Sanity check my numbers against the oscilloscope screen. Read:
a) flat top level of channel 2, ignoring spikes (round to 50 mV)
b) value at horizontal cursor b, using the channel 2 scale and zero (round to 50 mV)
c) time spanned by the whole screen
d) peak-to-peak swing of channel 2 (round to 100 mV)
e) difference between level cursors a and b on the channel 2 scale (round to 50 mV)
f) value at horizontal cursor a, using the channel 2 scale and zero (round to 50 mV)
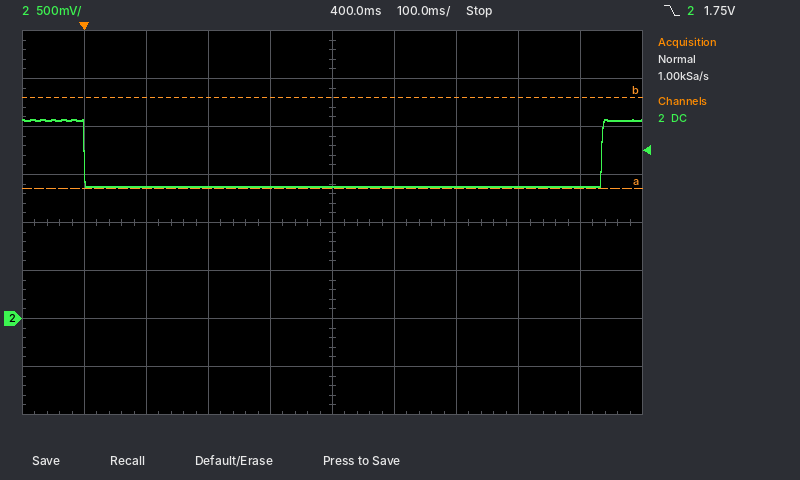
2.05 V
2.30 V
1 s
700 mV
950 mV
1.35 V
